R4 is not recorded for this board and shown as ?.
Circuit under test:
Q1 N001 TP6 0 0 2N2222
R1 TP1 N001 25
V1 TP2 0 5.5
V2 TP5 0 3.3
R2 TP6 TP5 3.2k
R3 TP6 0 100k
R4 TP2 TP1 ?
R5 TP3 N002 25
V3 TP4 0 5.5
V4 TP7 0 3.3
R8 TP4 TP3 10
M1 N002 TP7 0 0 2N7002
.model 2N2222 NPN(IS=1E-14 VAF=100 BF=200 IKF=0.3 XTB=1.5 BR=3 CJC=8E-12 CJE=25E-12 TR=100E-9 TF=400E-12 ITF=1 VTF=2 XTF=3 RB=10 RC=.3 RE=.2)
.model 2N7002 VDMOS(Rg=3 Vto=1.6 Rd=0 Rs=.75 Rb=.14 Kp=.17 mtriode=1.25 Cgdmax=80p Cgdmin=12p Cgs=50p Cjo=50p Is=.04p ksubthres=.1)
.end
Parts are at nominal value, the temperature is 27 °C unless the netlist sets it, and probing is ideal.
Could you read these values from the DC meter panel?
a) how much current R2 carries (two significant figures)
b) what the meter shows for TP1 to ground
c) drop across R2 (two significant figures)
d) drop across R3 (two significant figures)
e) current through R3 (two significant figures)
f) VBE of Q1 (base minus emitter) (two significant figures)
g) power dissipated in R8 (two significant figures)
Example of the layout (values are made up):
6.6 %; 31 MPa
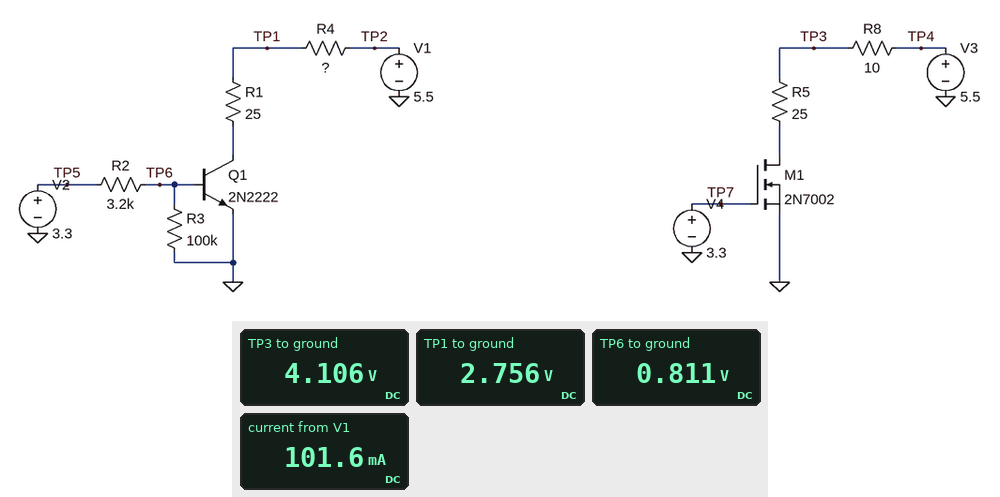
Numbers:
780 µA; 2.756 V; 2.5 V; 810 mV; 8.1 µA; 810 mV; 190 mW
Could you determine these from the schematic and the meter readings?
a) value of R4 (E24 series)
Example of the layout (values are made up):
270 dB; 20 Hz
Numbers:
27 Ω
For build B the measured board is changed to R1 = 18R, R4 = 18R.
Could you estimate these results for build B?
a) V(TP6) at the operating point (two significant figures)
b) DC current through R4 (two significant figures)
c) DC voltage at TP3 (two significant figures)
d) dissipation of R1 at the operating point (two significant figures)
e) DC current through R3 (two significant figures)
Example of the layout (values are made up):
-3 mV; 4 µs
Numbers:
820 mV; 110 mA; 4.1 V; 230 mW; 8.2 µA
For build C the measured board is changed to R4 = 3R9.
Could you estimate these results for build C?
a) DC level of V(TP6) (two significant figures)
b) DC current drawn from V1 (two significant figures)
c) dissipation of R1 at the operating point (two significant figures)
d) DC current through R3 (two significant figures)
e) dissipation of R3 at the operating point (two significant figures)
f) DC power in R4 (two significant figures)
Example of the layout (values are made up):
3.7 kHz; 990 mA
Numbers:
820 mV; 110 mA; 320 mW; 8.2 µA; 6.7 µW; 50 mW
